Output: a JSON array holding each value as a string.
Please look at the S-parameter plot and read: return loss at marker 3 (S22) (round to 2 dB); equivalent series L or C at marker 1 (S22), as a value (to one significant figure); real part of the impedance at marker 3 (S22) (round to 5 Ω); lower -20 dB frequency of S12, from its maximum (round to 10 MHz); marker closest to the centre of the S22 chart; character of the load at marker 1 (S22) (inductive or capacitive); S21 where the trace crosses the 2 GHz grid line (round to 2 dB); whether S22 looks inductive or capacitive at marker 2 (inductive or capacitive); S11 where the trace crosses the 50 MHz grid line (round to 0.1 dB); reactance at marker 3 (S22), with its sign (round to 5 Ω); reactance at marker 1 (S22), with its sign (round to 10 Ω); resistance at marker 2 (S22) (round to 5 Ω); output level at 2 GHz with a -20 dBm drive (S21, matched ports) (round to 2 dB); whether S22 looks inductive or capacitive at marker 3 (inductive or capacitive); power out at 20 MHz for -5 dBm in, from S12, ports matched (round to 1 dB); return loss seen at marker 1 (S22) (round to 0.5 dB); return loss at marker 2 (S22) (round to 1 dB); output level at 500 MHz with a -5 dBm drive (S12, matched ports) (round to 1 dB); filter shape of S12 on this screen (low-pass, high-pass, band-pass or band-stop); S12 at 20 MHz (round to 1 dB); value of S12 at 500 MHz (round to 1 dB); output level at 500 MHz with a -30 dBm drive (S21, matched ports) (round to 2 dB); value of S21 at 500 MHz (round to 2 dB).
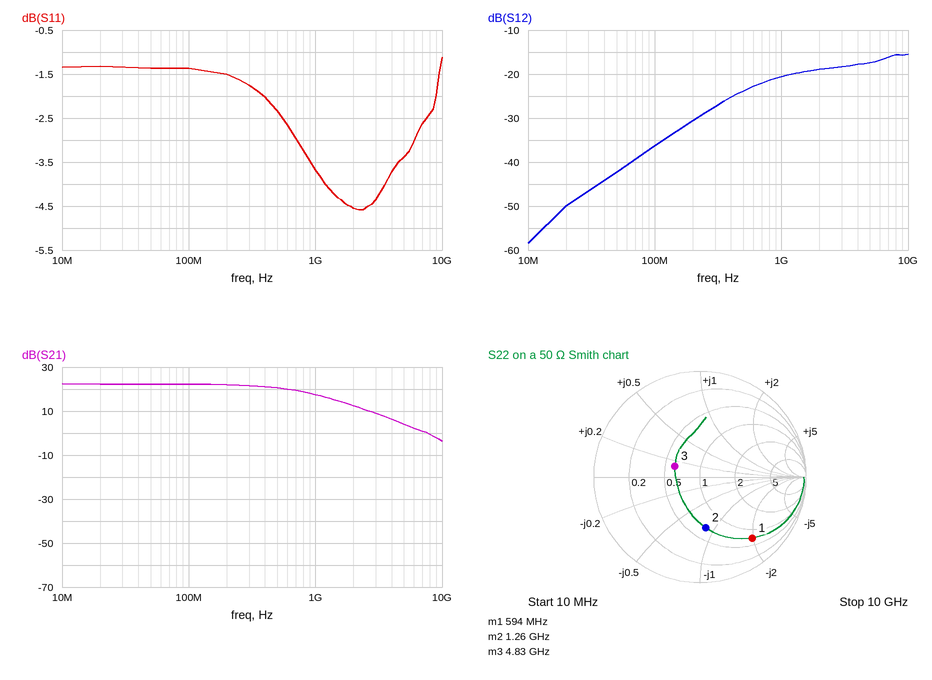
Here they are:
["12 dB", "3 pF", "30 Ω", "110 MHz", "marker 3", "capacitive", "12 dB", "capacitive", "-1.4 dB", "+5 Ω", "-100 Ω", "35 Ω", "-8 dBm", "inductive", "-55 dBm", "2.5 dB", "6 dB", "-29 dBm", "high-pass", "-50 dB", "-24 dB", "-10 dBm", "20 dB"]
